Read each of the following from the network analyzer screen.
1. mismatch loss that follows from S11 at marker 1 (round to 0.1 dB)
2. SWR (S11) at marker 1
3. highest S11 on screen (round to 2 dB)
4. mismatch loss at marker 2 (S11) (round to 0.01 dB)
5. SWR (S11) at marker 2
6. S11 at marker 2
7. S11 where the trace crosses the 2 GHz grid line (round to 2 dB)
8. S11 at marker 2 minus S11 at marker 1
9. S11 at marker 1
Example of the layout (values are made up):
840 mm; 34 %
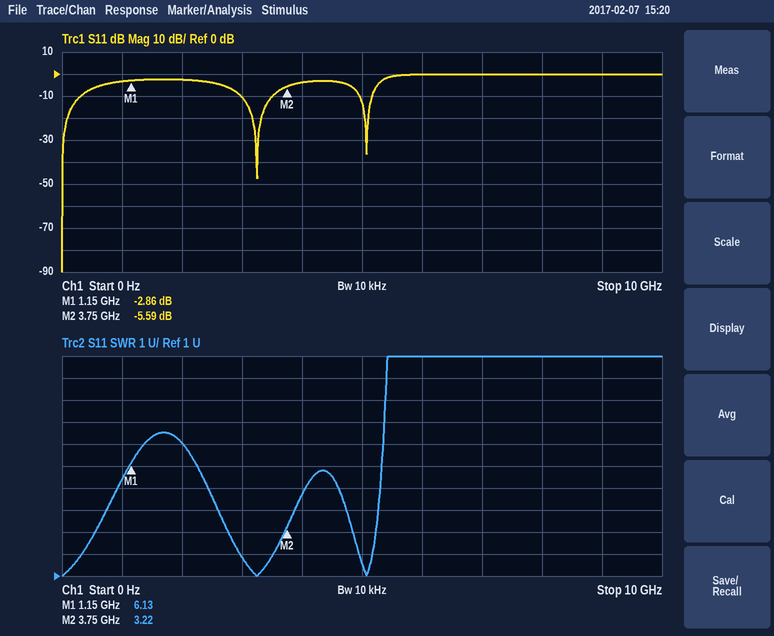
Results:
3.2 dB; 6.13; 0 dB; 1.40 dB; 3.22; -5.59 dB; -2 dB; -2.73 dB; -2.86 dB
